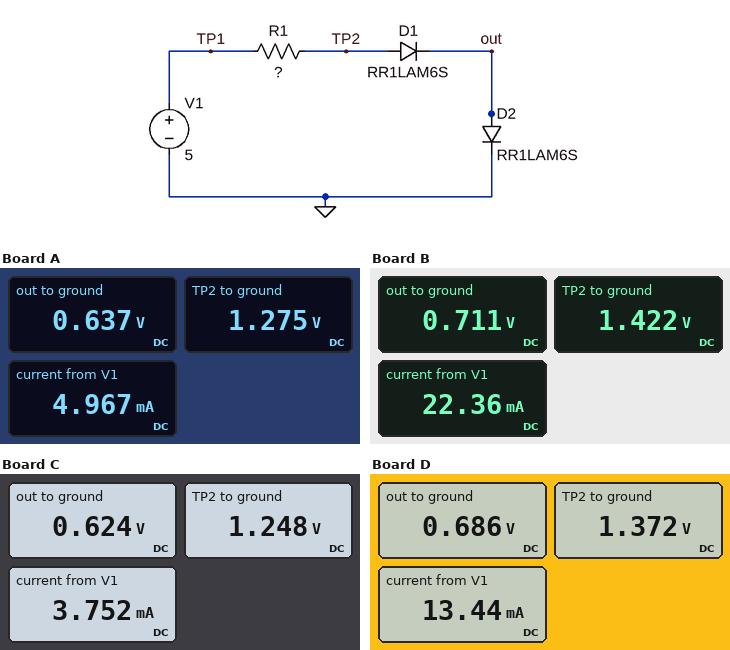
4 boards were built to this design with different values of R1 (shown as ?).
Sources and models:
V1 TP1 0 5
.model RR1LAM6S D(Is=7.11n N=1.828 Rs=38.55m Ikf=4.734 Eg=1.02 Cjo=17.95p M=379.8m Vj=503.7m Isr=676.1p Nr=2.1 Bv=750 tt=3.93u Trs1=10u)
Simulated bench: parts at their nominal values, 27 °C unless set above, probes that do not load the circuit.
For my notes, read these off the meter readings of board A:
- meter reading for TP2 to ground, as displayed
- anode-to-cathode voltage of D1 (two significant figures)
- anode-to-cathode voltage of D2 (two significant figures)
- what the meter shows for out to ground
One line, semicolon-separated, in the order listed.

1.275 V; 640 mV; 640 mV; 0.637 V
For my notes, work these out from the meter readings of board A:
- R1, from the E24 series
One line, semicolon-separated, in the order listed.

750 Ω
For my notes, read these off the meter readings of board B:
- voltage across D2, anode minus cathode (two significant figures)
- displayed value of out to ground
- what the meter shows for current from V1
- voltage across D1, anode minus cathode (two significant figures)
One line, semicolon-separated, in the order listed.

710 mV; 0.711 V; 22.36 mA; 710 mV
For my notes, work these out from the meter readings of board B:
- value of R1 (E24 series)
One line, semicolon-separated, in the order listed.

160 Ω
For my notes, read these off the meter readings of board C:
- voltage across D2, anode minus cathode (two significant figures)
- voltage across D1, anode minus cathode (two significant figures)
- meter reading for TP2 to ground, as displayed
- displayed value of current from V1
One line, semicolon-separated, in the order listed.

620 mV; 620 mV; 1.248 V; 3.752 mA
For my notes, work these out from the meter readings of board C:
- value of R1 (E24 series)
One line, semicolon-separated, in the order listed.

1 kΩ
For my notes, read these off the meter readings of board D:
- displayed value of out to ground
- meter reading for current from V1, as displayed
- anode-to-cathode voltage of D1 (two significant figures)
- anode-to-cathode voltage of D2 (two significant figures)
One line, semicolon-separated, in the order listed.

0.686 V; 13.44 mA; 690 mV; 690 mV
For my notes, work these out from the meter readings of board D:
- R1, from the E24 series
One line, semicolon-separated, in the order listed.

270 Ω
